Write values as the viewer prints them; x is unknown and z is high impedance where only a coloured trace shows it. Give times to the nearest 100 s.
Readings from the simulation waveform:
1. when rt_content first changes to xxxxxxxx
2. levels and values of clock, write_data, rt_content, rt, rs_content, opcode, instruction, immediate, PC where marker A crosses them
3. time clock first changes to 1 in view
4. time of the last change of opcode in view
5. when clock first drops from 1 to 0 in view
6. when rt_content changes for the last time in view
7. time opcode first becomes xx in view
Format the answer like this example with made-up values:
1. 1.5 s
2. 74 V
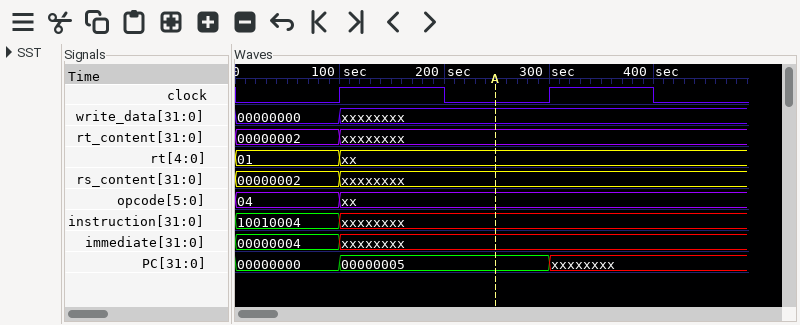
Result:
1. 100 s
2. clock=0, write_data=xxxxxxxx, rt_content=xxxxxxxx, rt=xx, rs_content=xxxxxxxx, opcode=xx, instruction=xxxxxxxx, immediate=xxxxxxxx, PC=00000005
3. 100 s
4. 100 s
5. 200 s
6. 100 s
7. 100 s
